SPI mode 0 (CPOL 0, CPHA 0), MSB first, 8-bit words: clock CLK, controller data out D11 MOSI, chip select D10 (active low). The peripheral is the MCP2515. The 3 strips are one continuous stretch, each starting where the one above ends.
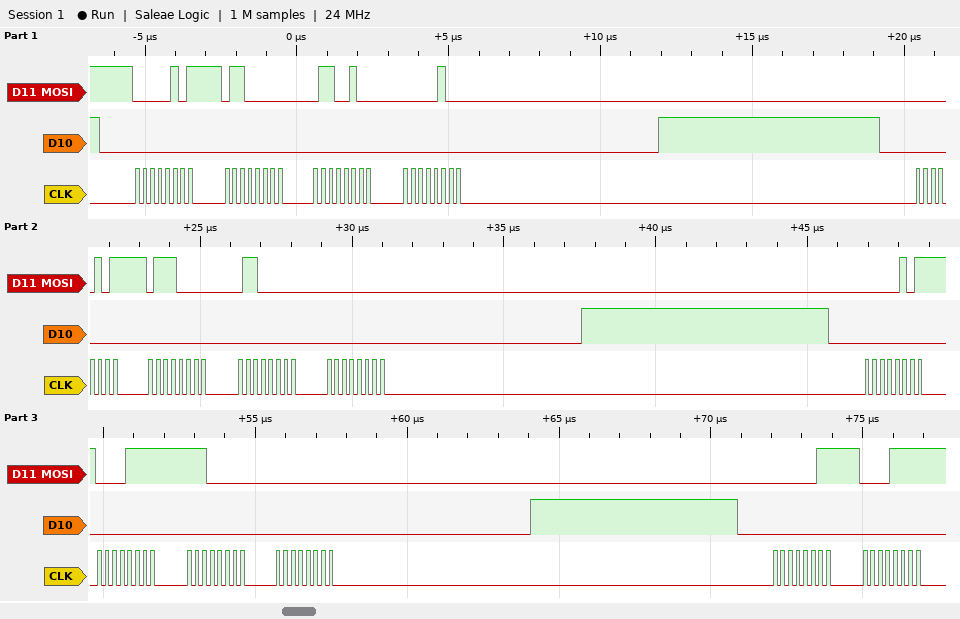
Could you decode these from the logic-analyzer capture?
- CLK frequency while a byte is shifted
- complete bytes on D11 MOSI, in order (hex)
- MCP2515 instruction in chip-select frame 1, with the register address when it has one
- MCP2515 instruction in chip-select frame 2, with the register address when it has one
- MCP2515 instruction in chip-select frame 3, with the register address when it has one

4 MHz
05 60 64 04 05 70 60 00 05 0F E0 00 03 0F
BIT MODIFY 0x60
BIT MODIFY 0x70
BIT MODIFY 0x0F
